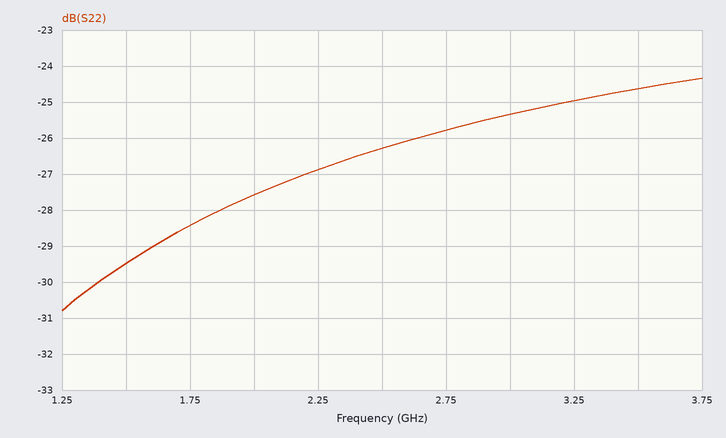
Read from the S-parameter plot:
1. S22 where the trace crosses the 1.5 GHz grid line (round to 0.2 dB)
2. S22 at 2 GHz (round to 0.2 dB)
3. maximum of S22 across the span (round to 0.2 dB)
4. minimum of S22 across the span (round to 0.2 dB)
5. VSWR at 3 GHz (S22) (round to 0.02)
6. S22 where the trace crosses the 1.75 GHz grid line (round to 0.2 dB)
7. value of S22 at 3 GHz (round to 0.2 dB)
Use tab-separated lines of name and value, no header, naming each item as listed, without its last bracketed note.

S22 where the trace crosses the 1.5 GHz grid line	-29.4 dB
S22 at 2 GHz	-27.6 dB
maximum of S22 across the span	-24.4 dB
minimum of S22 across the span	-30.8 dB
VSWR at 3 GHz (S22)	1.12
S22 where the trace crosses the 1.75 GHz grid line	-28.4 dB
value of S22 at 3 GHz	-25.4 dB
